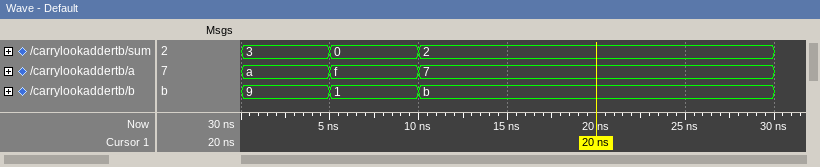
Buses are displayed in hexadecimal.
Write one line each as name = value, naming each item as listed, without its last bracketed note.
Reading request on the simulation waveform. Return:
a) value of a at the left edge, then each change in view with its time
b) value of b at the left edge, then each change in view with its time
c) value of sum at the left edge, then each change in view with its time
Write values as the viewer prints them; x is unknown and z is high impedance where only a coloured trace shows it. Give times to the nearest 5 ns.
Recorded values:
value of a at the left edge, then each change in view with its time = a, f at 5 ns, 7 at 10 ns
value of b at the left edge, then each change in view with its time = 9, 1 at 5 ns, b at 10 ns
value of sum at the left edge, then each change in view with its time = 3, 0 at 5 ns, 2 at 10 ns
